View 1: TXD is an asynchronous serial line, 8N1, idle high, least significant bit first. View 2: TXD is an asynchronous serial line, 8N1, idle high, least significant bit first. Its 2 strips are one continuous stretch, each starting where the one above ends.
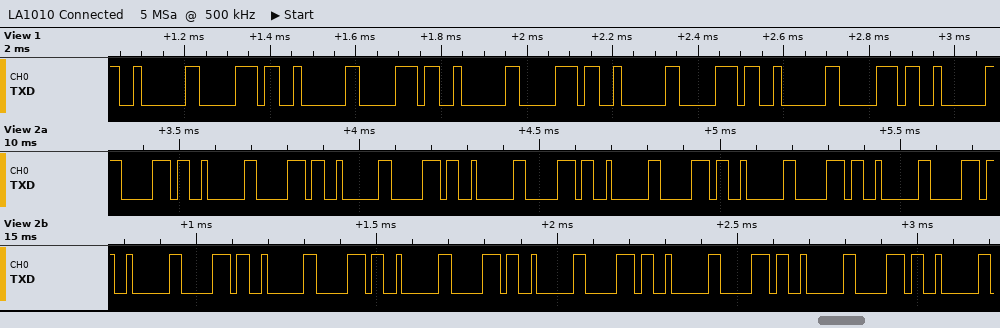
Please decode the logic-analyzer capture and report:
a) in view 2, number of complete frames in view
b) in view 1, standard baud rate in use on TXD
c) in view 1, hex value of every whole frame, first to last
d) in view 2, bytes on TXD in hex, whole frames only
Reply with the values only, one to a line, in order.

26
57600 baud
02 70 02 70 02 70 02 70 02 70 02
70 02 70 02 70 02 70 02 70 02 70 02 70 02 70 02 70 02 70 02 70 02 70 02 70 02
